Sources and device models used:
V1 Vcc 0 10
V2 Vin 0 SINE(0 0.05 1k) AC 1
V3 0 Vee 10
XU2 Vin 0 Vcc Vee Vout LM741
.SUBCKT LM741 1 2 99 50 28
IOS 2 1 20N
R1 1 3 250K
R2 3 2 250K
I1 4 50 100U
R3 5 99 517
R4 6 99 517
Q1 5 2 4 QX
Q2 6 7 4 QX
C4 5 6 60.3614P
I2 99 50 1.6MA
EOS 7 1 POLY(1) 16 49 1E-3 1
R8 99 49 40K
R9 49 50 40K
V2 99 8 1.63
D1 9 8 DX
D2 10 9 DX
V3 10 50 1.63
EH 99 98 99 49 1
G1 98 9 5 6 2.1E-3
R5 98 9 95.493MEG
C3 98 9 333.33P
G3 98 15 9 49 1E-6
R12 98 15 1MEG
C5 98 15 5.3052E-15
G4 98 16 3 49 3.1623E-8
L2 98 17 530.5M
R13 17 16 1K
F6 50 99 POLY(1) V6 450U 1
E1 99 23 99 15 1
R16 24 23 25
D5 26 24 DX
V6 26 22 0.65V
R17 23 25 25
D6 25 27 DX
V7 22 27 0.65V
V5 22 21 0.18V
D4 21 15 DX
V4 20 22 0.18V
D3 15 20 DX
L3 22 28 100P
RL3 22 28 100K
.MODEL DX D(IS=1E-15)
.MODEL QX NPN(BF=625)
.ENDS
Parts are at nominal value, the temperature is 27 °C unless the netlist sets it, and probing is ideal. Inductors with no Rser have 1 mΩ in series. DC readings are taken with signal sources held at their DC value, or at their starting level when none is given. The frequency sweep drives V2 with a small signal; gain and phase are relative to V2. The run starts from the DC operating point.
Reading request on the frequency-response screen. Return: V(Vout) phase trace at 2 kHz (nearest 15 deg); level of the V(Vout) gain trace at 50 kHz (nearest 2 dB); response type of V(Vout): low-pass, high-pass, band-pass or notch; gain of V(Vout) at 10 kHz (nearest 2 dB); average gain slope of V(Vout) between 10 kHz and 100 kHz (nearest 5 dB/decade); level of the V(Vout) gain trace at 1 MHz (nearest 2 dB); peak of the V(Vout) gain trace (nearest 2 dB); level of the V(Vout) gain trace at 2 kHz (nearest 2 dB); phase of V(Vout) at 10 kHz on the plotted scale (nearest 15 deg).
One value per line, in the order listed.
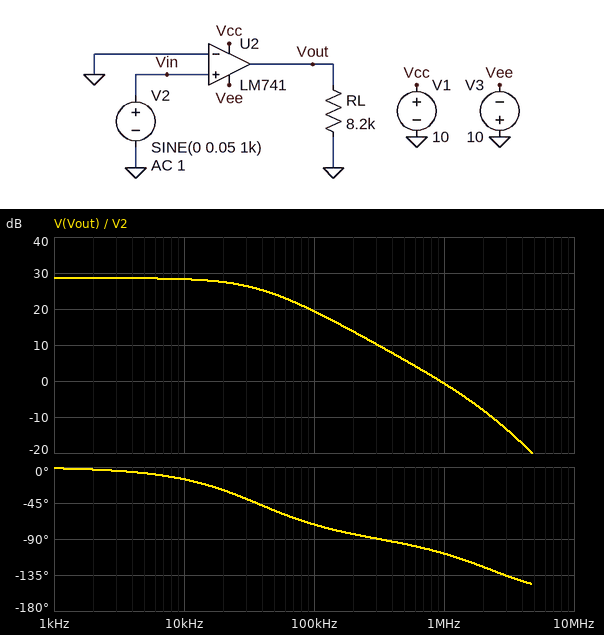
0 deg
24 dB
low-pass
28 dB
-10 dB/decade
0 dB
28 dB
28 dB
-15 deg
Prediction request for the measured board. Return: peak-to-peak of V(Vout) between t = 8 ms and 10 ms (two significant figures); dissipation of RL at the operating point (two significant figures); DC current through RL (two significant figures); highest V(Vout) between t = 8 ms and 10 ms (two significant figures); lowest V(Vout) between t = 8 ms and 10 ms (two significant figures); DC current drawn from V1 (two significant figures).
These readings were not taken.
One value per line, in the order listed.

18 V
9.5 mW
1.1 mA
8.9 V
-8.9 V
2.6 mA
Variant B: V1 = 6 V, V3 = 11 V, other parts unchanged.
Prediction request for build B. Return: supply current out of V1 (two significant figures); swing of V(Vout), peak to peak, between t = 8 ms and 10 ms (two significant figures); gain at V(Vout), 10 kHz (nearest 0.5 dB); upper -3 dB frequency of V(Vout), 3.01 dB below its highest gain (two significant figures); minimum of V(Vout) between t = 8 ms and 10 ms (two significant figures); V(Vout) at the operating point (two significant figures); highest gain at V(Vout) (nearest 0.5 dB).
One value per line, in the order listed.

2.1 mA
15 V
27.5 dB
40 kHz
-9.9 V
4.9 V
28.0 dB
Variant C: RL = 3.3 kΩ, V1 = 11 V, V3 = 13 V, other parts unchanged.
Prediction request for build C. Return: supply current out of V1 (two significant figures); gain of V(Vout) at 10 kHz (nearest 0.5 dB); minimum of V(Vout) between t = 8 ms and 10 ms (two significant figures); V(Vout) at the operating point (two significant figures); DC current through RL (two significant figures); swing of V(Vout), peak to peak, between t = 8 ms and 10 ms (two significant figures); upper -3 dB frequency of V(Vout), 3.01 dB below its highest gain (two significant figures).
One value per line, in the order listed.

4.5 mA
28.0 dB
-12 V
9.8 V
3.0 mA
22 V
38 kHz
